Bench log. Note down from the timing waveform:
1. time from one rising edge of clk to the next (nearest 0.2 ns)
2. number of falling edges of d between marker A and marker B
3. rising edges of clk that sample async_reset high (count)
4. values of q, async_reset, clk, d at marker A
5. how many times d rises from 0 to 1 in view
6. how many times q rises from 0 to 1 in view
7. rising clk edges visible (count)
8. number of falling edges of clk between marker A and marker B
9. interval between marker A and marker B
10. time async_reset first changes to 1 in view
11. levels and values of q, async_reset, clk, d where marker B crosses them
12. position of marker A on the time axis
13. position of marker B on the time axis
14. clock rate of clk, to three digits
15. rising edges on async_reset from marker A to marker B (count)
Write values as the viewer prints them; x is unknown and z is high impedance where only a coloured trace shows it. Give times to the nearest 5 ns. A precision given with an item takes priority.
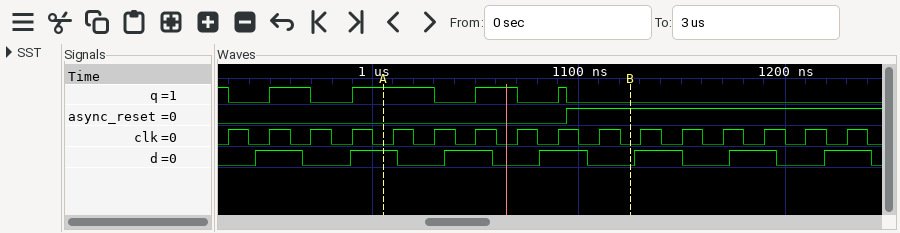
20 ns
3
7
q=1, async_reset=0, clk=0, d=1
7
4
16
6
120 ns
1095 ns
q=0, async_reset=1, clk=0, d=0
1005 ns
1125 ns
50.0 MHz
1
